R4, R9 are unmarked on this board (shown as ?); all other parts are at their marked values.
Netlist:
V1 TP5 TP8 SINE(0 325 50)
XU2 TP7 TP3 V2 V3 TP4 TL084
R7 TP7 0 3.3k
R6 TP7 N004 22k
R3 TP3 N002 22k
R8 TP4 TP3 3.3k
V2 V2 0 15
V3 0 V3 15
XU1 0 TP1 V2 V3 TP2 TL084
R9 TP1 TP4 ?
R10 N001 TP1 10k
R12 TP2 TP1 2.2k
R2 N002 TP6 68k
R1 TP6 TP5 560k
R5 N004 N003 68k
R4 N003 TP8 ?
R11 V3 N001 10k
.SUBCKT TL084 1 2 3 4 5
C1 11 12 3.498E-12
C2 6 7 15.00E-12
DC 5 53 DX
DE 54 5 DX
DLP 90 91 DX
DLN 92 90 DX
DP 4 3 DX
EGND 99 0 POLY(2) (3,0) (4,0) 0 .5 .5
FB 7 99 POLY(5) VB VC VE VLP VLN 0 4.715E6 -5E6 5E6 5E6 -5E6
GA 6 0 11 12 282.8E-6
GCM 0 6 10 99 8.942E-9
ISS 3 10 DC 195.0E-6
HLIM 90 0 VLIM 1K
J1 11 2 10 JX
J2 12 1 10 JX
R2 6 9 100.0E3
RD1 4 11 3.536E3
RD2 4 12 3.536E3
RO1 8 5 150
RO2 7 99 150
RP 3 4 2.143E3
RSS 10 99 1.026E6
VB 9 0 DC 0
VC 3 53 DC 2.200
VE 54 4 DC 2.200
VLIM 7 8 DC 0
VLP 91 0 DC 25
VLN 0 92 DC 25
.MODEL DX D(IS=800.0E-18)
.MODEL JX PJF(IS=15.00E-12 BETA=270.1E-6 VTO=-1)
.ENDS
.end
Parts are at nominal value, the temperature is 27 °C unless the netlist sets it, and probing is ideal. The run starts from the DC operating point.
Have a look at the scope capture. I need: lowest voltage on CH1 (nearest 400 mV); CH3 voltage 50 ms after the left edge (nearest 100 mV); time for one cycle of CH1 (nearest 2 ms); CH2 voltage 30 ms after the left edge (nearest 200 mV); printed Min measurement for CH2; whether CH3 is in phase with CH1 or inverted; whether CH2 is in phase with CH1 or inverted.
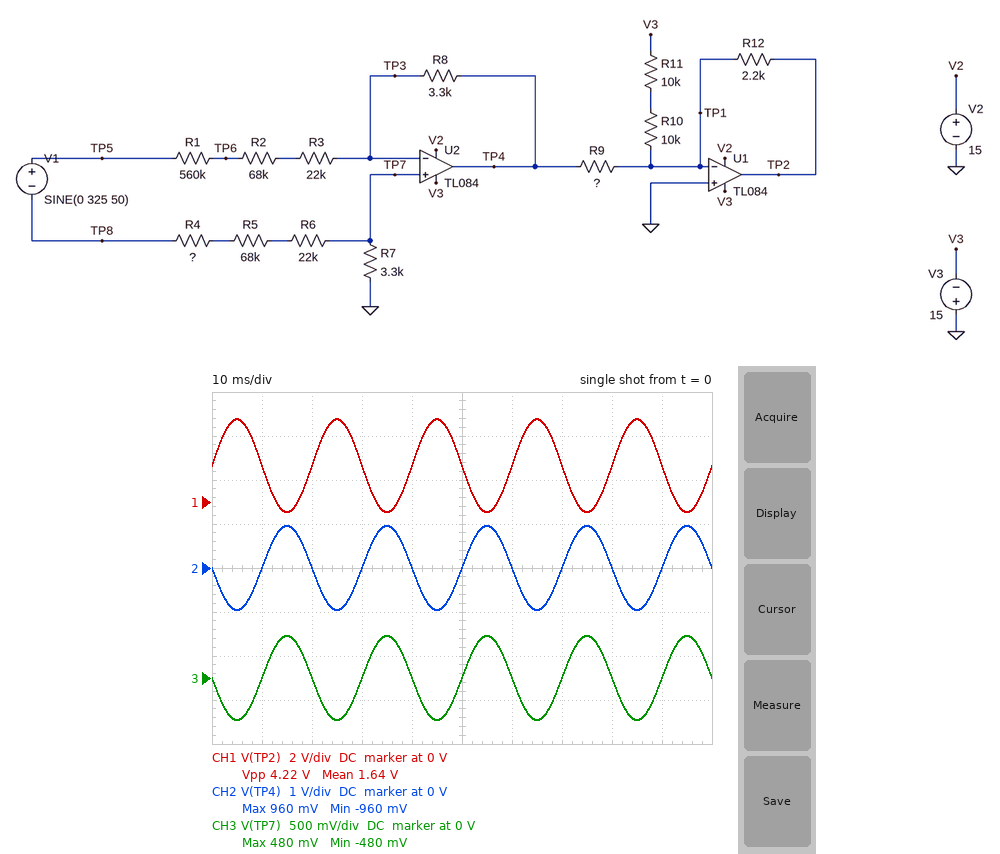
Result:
-400 mV
0 V
20 ms
0 V
-960 mV
inverted
inverted
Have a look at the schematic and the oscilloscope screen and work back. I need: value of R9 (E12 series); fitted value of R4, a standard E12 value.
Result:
1 kΩ
1.5 MΩ
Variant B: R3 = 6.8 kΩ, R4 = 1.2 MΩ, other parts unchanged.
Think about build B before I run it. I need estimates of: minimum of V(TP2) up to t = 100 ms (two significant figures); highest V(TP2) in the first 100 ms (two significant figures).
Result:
-800 mV
4.1 V
